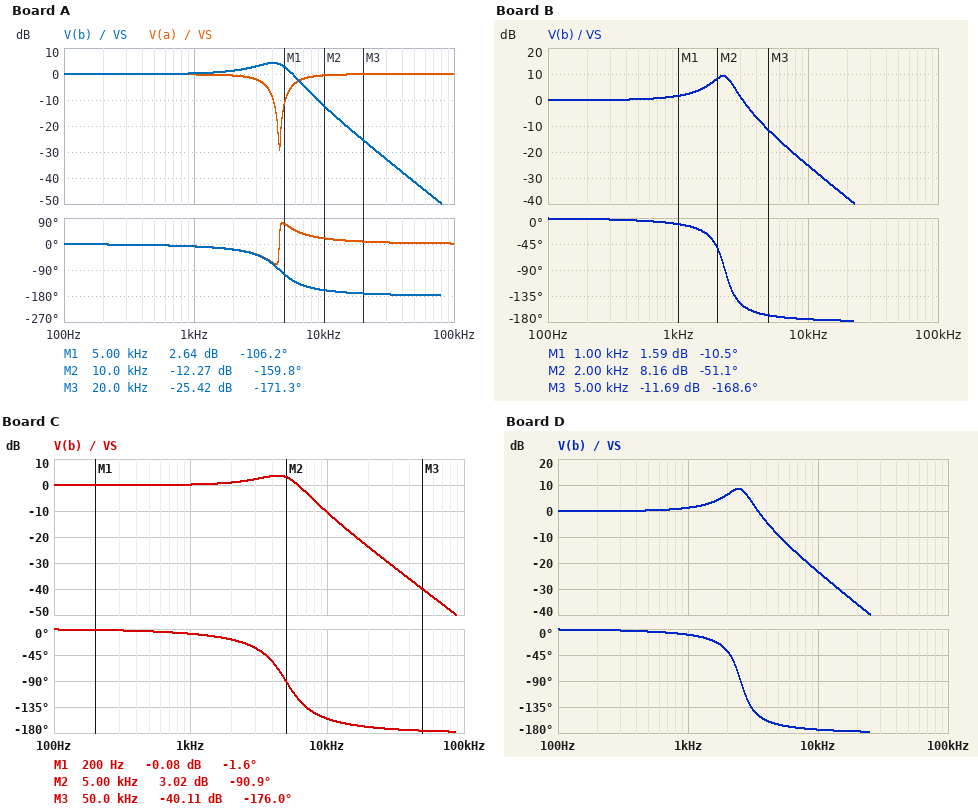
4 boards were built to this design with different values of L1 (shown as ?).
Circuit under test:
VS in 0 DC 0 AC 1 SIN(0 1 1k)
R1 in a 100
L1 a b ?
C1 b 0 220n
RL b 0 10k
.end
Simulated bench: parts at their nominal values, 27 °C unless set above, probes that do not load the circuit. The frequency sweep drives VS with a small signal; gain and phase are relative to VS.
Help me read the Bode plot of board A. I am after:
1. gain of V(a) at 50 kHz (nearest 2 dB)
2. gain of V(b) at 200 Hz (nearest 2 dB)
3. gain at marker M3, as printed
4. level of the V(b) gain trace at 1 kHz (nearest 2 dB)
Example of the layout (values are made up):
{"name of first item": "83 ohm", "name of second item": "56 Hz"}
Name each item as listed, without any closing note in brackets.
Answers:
{"gain of V(a) at 50 kHz": "0 dB", "gain of V(b) at 200 Hz": "0 dB", "gain at marker M3, as printed": "-25.42 dB", "level of the V(b) gain trace at 1 kHz": "0 dB"}
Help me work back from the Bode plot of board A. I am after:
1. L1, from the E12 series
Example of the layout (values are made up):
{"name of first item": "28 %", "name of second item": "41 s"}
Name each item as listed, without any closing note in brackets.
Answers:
{"L1, from the E12 series": "5.6 mH"}
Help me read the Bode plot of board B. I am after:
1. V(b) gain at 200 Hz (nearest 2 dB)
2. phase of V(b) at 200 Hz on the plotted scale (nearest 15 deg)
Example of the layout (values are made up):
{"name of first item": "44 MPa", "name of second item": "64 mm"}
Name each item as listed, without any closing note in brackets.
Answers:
{"V(b) gain at 200 Hz": "0 dB", "phase of V(b) at 200 Hz on the plotted scale": "0 deg"}
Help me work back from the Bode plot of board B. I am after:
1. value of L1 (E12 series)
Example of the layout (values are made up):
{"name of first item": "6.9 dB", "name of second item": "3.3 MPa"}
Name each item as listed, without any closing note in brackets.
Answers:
{"value of L1": "22 mH"}
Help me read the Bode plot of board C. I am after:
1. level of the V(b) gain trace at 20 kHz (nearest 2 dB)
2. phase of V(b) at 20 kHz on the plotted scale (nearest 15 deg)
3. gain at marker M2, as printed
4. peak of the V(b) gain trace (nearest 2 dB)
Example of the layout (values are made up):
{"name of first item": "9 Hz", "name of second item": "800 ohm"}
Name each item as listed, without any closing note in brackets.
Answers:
{"level of the V(b) gain trace at 20 kHz": "-24 dB", "phase of V(b) at 20 kHz on the plotted scale": "-165 deg", "gain at marker M2, as printed": "3.02 dB", "peak of the V(b) gain trace": "4 dB"}
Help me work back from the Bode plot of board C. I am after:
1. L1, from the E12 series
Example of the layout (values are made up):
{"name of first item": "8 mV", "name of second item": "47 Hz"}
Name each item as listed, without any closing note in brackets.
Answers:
{"L1, from the E12 series": "4.7 mH"}
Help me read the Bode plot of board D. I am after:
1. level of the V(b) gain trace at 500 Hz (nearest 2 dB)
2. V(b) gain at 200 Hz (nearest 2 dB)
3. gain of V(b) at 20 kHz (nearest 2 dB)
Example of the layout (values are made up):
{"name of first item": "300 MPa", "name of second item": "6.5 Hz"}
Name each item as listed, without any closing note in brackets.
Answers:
{"level of the V(b) gain trace at 500 Hz": "0 dB", "V(b) gain at 200 Hz": "0 dB", "gain of V(b) at 20 kHz": "-36 dB"}
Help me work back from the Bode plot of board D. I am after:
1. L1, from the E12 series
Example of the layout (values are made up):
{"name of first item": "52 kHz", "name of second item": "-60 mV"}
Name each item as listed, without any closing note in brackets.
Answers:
{"L1, from the E12 series": "18 mH"}
